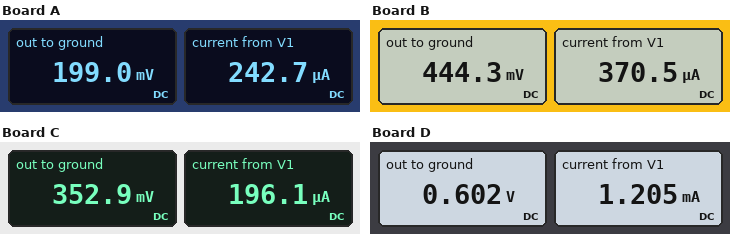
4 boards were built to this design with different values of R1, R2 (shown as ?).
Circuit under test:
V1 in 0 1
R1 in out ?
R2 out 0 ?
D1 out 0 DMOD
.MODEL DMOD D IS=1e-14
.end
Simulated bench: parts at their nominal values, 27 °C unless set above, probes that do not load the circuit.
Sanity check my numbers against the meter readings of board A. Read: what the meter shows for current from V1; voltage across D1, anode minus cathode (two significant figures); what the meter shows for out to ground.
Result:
242.7 µA
200 mV
199.0 mV
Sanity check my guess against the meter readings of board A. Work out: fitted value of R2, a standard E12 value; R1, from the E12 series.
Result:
820 Ω
3.3 kΩ
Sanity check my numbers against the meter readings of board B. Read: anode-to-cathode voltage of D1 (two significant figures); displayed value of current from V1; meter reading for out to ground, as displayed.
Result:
440 mV
370.5 µA
444.3 mV
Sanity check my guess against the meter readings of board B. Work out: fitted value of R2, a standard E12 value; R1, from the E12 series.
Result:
1.2 kΩ
1.5 kΩ
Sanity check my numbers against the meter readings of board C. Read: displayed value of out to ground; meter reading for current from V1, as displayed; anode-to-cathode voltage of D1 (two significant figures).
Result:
352.9 mV
196.1 µA
350 mV
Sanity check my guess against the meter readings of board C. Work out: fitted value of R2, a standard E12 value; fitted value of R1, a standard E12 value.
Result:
1.8 kΩ
3.3 kΩ
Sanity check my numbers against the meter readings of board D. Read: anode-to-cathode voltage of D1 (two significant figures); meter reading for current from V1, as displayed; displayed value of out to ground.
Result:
600 mV
1.205 mA
0.602 V
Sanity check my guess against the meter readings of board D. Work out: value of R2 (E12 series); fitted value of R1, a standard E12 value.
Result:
560 Ω
330 Ω
